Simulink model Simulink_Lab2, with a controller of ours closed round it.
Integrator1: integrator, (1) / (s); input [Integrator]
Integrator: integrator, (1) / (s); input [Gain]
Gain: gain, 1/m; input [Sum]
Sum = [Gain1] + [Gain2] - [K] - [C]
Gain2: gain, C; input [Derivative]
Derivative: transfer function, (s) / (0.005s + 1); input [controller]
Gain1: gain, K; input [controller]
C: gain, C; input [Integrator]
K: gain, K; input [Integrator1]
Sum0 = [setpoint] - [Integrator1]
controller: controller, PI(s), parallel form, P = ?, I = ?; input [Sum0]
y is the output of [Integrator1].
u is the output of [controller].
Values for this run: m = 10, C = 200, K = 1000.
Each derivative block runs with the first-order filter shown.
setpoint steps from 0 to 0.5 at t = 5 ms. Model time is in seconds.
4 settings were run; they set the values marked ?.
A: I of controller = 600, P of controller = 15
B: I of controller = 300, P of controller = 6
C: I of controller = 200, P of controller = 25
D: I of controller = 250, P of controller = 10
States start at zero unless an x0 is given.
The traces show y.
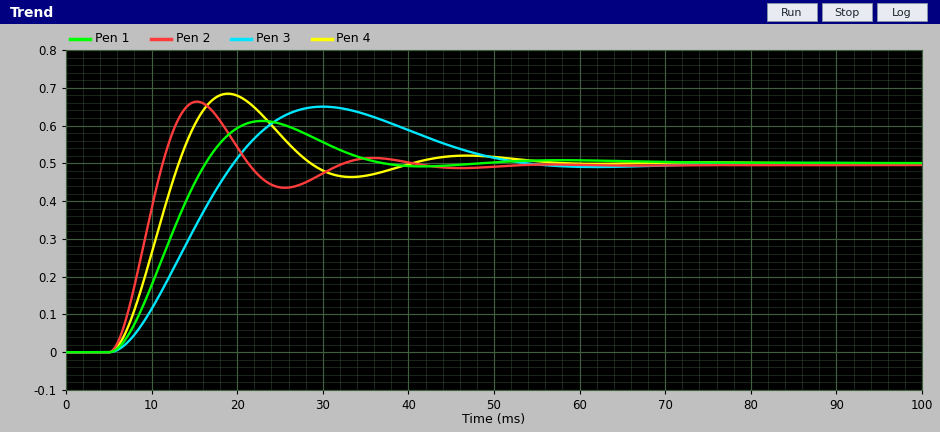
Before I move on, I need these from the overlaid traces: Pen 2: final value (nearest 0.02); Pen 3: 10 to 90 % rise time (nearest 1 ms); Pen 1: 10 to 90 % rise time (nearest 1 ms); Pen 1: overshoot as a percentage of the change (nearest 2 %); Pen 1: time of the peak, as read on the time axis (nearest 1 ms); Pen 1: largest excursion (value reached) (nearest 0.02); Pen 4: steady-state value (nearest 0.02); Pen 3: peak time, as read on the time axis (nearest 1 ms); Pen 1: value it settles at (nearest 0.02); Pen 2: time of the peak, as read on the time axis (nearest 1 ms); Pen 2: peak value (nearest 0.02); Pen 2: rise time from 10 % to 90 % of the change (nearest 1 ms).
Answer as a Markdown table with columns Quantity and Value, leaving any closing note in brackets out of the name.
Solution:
| Quantity | Value |
|---|---|
| Pen 2: final value | 0.50 |
| Pen 3: 10 to 90 % rise time | 10 ms |
| Pen 1: 10 to 90 % rise time | 8 ms |
| Pen 1: overshoot as a percentage of the change | 22 % |
| Pen 1: time of the peak, as read on the time axis | 23 ms |
| Pen 1: largest excursion (value reached) | 0.62 |
| Pen 4: steady-state value | 0.50 |
| Pen 3: peak time, as read on the time axis | 30 ms |
| Pen 1: value it settles at | 0.50 |
| Pen 2: time of the peak, as read on the time axis | 15 ms |
| Pen 2: peak value | 0.66 |
| Pen 2: rise time from 10 % to 90 % of the change | 4 ms |
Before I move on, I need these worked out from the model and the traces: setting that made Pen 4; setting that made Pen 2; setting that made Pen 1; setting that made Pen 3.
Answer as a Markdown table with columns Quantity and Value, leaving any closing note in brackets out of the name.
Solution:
| Quantity | Value |
|---|---|
| setting that made Pen 4 | A |
| setting that made Pen 2 | C |
| setting that made Pen 1 | D |
| setting that made Pen 3 | B |
